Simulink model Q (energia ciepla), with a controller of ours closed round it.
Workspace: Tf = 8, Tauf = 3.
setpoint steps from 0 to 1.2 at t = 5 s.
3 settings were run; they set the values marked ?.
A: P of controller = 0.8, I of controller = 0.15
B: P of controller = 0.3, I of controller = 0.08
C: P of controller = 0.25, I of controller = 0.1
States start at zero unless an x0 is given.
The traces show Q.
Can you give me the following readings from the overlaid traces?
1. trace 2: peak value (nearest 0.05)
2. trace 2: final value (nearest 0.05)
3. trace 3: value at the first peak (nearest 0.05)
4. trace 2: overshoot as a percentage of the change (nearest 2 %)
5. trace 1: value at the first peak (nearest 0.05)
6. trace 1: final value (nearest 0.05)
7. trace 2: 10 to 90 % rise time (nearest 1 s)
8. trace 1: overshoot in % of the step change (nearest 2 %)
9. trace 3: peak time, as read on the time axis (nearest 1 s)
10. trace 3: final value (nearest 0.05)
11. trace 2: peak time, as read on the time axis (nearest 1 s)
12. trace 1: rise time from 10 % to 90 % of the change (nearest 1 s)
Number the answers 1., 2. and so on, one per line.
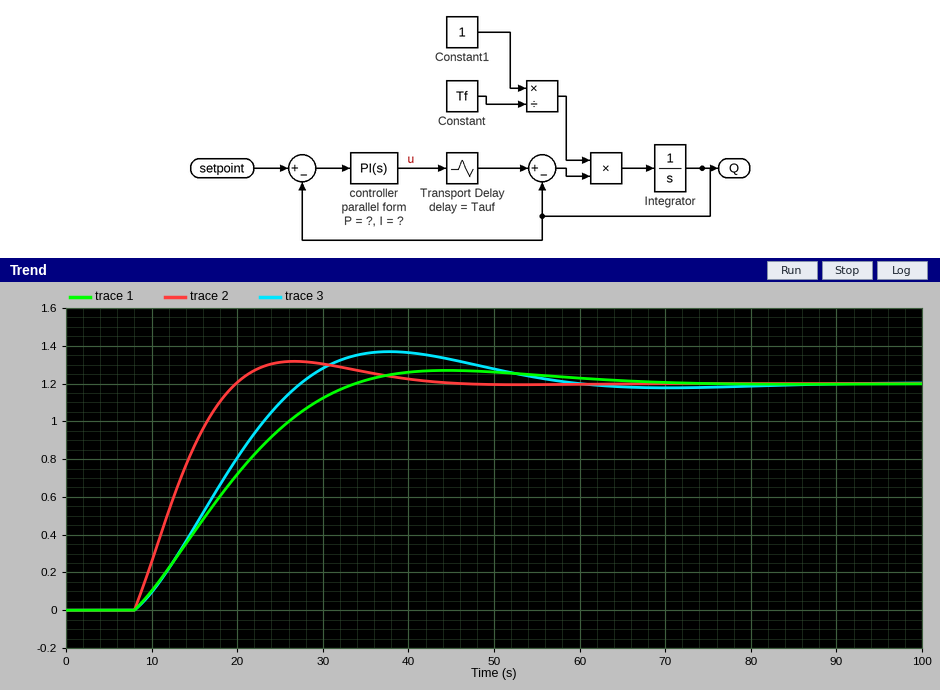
1. 1.30
2. 1.20
3. 1.35
4. 10 %
5. 1.25
6. 1.20
7. 9 s
8. 6 %
9. 38 s
10. 1.20
11. 27 s
12. 18 s
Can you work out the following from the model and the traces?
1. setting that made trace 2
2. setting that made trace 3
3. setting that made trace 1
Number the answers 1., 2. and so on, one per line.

1. A
2. C
3. B
